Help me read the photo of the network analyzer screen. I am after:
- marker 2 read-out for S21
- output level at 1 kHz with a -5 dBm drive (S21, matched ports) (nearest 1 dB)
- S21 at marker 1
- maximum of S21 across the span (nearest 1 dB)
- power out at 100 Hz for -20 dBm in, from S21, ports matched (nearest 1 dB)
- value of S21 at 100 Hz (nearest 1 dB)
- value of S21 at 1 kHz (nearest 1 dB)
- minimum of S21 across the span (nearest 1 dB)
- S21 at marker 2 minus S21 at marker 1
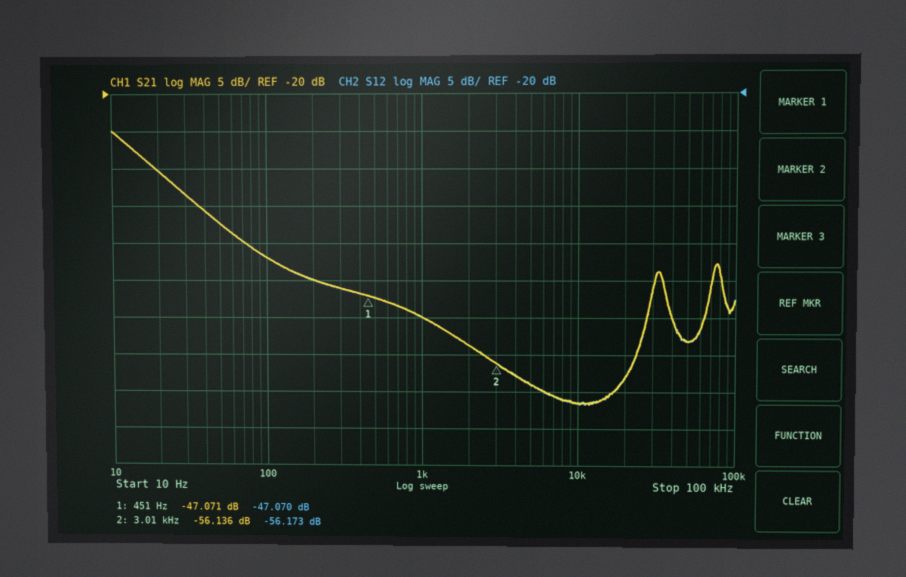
-56.136 dB
-55 dBm
-47.071 dB
-25 dB
-62 dBm
-42 dB
-50 dB
-62 dB
-9.065 dB
